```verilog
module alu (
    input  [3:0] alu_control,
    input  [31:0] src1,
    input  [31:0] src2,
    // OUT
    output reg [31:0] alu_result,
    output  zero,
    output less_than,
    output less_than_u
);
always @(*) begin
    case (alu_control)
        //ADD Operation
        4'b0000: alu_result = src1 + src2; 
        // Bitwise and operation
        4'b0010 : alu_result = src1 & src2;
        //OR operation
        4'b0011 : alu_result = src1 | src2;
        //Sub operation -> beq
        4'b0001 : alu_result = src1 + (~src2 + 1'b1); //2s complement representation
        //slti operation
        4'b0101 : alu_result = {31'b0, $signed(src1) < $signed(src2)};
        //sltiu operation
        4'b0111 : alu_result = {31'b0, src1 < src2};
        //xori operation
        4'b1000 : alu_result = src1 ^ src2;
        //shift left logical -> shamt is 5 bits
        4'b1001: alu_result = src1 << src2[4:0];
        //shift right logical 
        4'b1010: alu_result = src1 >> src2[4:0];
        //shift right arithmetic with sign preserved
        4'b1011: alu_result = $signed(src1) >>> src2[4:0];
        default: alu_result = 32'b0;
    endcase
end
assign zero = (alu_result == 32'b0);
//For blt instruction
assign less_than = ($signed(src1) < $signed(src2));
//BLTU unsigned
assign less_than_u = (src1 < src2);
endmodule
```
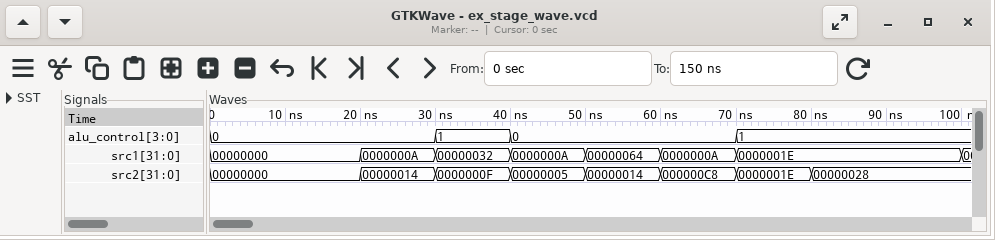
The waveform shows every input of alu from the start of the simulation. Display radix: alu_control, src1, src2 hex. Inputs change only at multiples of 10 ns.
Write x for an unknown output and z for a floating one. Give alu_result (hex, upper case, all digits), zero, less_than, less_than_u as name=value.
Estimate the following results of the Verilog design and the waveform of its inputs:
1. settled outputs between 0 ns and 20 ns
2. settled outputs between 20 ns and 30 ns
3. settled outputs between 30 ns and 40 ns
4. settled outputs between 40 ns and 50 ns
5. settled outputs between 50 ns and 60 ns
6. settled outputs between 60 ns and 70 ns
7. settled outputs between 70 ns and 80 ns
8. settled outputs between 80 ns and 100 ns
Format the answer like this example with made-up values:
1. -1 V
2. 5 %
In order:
1. alu_result=00000000, zero=1, less_than=0, less_than_u=0
2. alu_result=0000001E, zero=0, less_than=1, less_than_u=1
3. alu_result=00000023, zero=0, less_than=0, less_than_u=0
4. alu_result=0000000F, zero=0, less_than=0, less_than_u=0
5. alu_result=00000078, zero=0, less_than=0, less_than_u=0
6. alu_result=000000D2, zero=0, less_than=1, less_than_u=1
7. alu_result=00000000, zero=1, less_than=0, less_than_u=0
8. alu_result=FFFFFFF6, zero=0, less_than=1, less_than_u=1
